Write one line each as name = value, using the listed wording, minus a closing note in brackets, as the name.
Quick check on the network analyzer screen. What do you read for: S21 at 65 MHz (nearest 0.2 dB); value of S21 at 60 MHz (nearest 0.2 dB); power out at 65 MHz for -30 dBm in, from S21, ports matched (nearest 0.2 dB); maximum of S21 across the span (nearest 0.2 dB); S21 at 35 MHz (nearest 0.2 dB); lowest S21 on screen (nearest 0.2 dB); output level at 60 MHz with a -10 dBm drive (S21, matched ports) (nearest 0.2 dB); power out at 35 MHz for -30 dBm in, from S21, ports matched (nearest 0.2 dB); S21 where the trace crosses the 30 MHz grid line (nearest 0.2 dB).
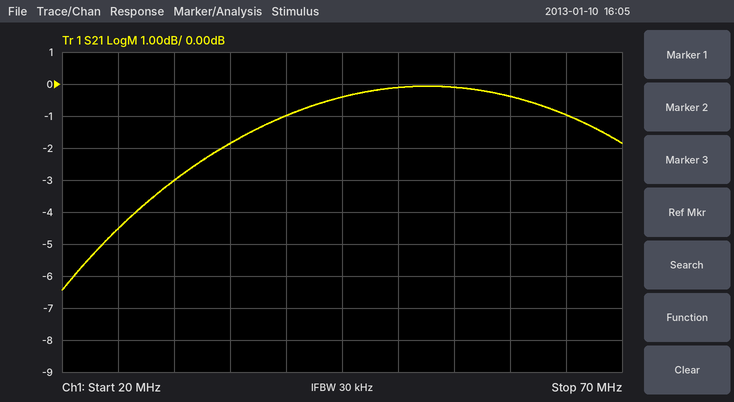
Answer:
S21 at 65 MHz = -1.0 dB
value of S21 at 60 MHz = -0.4 dB
power out at 65 MHz for -30 dBm in, from S21, ports matched = -31.0 dBm
maximum of S21 across the span = 0.0 dB
S21 at 35 MHz = -1.8 dB
lowest S21 on screen = -6.4 dB
output level at 60 MHz with a -10 dBm drive (S21, matched ports) = -10.4 dBm
power out at 35 MHz for -30 dBm in, from S21, ports matched = -31.8 dBm
S21 where the trace crosses the 30 MHz grid line = -3.0 dB
